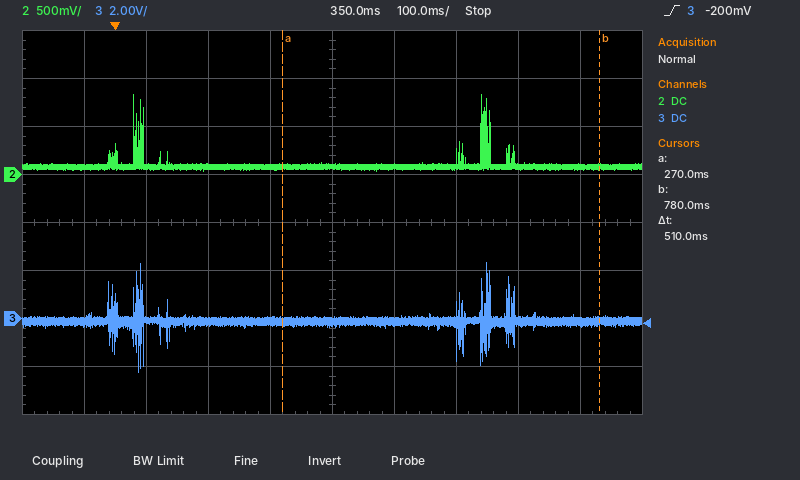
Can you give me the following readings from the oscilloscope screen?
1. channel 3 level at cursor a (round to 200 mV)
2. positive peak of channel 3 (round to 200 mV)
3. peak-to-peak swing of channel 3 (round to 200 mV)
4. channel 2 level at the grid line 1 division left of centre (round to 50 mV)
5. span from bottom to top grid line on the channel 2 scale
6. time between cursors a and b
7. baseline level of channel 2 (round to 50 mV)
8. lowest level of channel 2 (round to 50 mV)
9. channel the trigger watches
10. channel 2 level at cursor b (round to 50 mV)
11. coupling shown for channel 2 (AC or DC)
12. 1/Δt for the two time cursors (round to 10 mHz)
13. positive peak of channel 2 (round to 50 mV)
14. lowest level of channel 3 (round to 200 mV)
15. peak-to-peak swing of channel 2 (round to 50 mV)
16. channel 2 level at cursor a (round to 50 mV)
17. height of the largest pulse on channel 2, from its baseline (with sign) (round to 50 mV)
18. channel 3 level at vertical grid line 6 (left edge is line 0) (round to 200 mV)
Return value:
-200 mV
2.4 V
4.6 V
100 mV
4 V
510 ms
100 mV
50 mV
channel 3
100 mV
DC
1.96 Hz
850 mV
-2.2 V
800 mV
100 mV
+750 mV
-200 mV
